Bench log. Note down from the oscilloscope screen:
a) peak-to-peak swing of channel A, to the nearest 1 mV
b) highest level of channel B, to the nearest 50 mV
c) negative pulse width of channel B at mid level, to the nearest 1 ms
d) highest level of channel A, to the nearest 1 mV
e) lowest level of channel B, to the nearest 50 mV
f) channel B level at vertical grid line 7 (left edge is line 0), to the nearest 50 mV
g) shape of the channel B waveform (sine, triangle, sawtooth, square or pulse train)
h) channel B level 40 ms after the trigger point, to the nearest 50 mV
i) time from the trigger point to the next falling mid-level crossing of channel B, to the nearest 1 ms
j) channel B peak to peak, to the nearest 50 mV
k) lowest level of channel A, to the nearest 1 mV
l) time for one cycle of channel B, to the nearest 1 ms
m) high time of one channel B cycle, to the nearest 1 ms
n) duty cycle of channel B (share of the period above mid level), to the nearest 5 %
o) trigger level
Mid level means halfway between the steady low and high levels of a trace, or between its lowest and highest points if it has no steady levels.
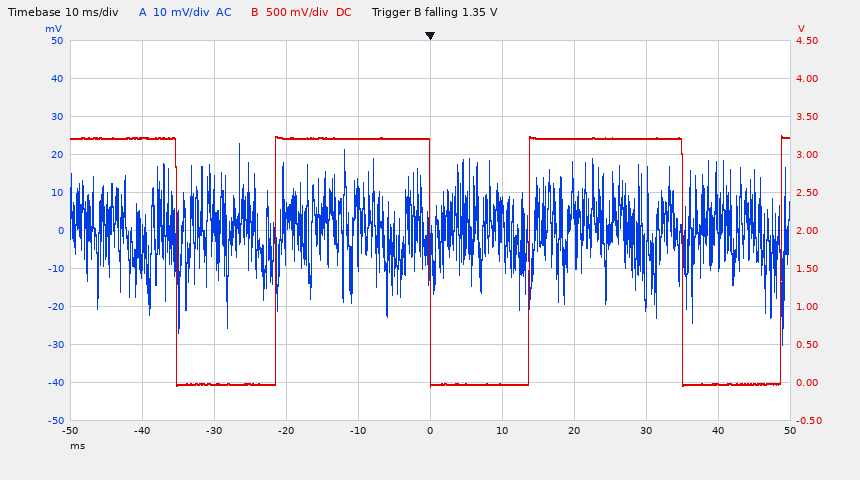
53 mV
3.25 V
14 ms
23 mV
-50 mV
3.20 V
pulse train
0 mV
35 ms
3.30 V
-30 mV
35 ms
21 ms
60 %
1.35 V
